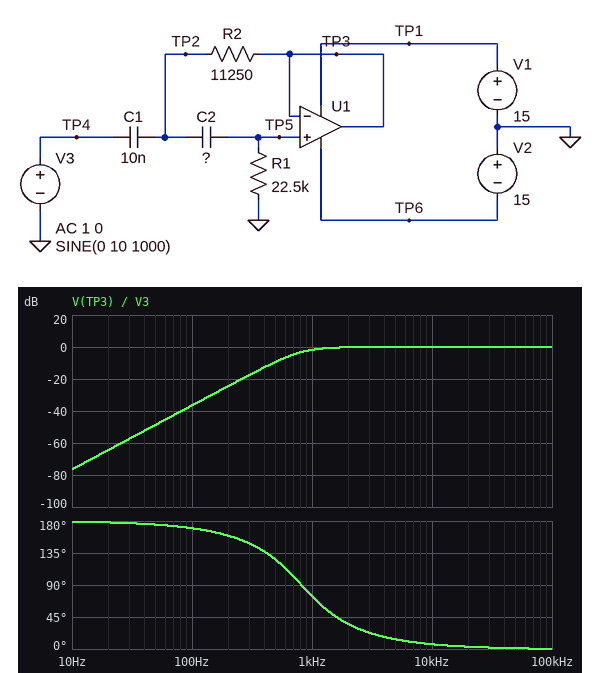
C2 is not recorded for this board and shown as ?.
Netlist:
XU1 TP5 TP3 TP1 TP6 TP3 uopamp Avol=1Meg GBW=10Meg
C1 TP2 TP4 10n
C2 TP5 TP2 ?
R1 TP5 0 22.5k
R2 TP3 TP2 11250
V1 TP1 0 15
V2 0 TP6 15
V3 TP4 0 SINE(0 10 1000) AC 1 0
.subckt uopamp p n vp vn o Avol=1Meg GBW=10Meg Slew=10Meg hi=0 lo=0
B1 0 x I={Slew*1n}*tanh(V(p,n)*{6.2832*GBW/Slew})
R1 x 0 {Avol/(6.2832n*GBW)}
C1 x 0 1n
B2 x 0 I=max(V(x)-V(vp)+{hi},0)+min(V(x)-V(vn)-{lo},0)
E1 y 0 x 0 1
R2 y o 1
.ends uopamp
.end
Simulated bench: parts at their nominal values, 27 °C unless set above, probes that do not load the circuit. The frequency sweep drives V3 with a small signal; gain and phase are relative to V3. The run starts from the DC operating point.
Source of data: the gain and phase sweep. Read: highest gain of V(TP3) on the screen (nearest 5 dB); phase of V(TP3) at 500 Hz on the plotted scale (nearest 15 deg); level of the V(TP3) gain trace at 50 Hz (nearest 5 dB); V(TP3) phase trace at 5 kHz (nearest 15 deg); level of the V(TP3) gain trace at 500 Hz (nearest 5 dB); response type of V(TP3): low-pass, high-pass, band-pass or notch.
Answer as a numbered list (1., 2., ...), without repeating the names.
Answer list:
1. 0 dB
2. 120 deg
3. -50 dB
4. 15 deg
5. -10 dB
6. high-pass
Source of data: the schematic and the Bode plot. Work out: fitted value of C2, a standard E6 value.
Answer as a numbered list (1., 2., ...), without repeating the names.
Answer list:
1. 15 nF
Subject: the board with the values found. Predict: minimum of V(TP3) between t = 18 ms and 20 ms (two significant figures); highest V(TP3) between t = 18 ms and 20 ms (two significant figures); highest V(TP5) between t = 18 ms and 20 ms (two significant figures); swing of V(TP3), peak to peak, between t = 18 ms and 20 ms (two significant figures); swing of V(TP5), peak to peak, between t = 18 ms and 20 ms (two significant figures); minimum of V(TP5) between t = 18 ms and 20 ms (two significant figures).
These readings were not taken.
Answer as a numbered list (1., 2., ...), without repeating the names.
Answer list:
1. -8.2 V
2. 8.2 V
3. 8.2 V
4. 16 V
5. 16 V
6. -8.2 V
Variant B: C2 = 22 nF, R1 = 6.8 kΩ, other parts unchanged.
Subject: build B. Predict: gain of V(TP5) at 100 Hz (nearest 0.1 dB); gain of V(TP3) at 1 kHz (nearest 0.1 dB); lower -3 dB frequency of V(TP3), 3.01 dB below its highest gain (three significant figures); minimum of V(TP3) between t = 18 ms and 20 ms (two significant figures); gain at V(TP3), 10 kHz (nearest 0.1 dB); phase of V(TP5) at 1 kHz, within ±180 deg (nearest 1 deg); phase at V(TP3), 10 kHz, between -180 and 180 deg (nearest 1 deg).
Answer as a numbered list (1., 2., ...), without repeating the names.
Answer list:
1. -43.7 dB
2. -10.7 dB
3. 2.97 kHz
4. -2.9 V
5. -0.4 dB
6. 98 deg
7. 19 deg
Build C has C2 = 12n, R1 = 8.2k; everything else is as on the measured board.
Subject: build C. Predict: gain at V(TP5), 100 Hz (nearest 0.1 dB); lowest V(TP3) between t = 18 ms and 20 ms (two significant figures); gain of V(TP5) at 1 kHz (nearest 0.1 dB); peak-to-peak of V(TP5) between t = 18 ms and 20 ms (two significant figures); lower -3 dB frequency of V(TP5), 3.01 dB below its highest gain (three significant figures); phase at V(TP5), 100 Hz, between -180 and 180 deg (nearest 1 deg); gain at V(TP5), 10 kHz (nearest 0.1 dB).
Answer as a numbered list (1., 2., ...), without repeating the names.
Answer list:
1. -47.3 dB
2. -2.6 V
3. -11.6 dB
4. 5.3 V
5. 2.95 kHz
6. 171 deg
7. -0.3 dB
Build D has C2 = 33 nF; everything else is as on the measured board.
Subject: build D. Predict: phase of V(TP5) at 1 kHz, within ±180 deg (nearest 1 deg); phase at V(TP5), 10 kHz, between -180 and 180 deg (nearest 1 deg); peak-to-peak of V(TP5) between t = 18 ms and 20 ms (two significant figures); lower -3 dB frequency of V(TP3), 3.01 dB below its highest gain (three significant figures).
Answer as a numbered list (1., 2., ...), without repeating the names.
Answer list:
1. 53 deg
2. 5 deg
3. 17 V
4. 669 Hz
